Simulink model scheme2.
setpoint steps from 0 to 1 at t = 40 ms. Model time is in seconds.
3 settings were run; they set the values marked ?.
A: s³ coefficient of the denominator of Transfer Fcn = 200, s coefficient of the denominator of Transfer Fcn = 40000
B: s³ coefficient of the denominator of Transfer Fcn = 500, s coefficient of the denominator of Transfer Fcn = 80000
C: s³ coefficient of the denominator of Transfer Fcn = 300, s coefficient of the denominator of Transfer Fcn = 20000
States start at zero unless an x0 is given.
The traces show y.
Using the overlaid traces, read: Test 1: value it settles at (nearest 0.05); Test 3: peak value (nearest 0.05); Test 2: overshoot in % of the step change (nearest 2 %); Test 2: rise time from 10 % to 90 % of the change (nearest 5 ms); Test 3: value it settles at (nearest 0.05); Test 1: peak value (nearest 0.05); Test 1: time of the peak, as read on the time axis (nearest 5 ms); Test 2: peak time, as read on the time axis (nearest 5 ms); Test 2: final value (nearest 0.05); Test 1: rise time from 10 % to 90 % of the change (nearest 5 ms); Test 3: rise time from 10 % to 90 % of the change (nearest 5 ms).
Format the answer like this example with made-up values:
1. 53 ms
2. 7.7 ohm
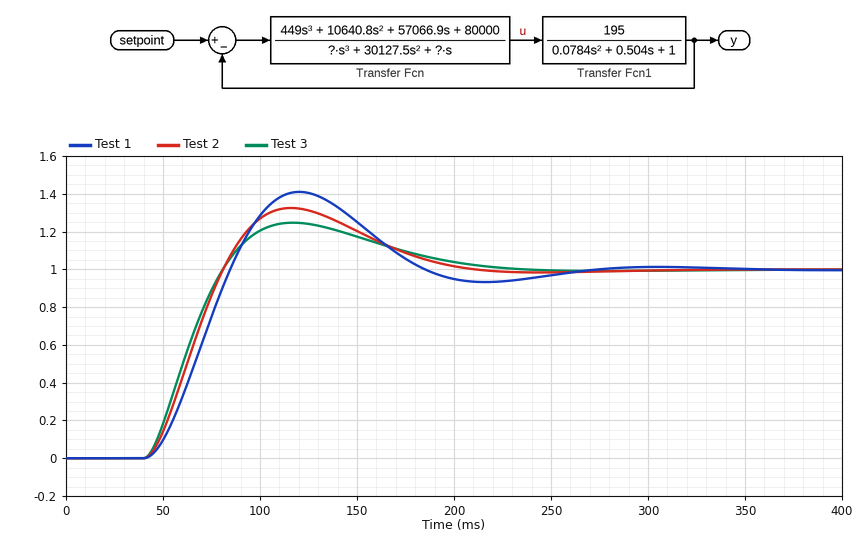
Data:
1. 1.00
2. 1.25
3. 32 %
4. 30 ms
5. 1.00
6. 1.40
7. 120 ms
8. 115 ms
9. 1.00
10. 30 ms
11. 30 ms
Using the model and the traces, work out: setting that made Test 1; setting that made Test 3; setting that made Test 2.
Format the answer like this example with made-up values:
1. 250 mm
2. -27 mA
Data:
1. B
2. A
3. C
